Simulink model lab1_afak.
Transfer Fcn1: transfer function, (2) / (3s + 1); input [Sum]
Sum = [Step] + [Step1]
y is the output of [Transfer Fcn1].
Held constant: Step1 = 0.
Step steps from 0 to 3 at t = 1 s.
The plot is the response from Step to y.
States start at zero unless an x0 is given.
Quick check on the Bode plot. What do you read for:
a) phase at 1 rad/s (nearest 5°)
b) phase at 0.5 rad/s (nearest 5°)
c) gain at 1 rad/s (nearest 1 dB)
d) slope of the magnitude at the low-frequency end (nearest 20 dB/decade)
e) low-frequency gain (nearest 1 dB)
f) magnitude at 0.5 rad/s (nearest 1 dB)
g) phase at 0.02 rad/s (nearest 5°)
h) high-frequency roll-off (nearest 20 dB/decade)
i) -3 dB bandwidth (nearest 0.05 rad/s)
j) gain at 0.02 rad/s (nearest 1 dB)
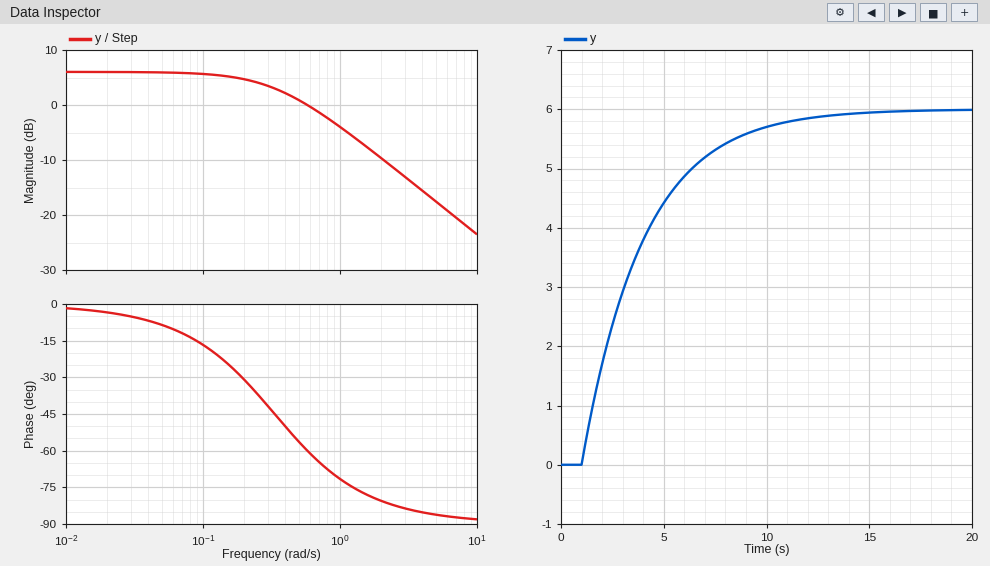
-70°
-55°
-4 dB
0 dB/decade
6 dB
1 dB
-5°
-20 dB/decade
0.35 rad/s
6 dB
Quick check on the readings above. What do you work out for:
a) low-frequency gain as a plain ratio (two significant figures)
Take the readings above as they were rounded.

2.0
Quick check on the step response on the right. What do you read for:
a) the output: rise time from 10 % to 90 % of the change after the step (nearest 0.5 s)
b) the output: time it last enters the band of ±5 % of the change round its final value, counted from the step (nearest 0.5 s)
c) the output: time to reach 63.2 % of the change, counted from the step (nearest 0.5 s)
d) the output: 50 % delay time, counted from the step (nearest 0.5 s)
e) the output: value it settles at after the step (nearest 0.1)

6.5 s
9.0 s
3.0 s
2.0 s
6.0
